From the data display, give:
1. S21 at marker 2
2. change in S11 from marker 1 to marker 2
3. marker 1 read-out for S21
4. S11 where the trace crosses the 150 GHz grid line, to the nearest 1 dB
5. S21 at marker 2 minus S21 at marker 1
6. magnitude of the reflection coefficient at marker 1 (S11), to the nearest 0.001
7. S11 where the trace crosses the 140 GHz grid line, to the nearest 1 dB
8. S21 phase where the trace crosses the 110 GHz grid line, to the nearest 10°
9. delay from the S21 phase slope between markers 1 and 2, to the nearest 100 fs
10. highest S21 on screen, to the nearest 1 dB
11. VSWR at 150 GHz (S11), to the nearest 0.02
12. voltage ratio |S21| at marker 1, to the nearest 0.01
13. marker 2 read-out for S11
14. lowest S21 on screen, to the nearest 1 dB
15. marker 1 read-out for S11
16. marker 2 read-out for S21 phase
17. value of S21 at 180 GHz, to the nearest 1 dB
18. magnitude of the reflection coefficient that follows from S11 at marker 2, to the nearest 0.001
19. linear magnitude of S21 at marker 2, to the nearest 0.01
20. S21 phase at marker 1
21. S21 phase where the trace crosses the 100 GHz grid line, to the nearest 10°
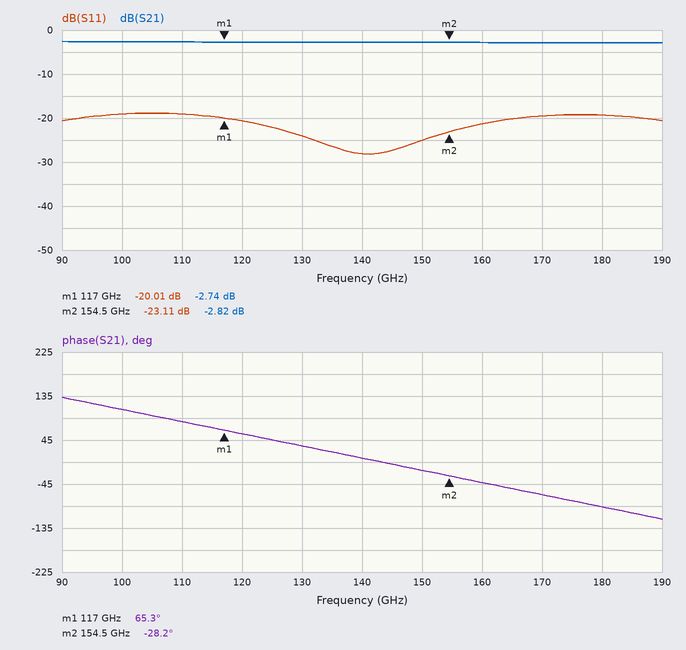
-2.82 dB
-3.10 dB
-2.74 dB
-25 dB
-0.08 dB
0.100
-28 dB
80°
6.9 ps
-3 dB
1.12
0.73
-23.11 dB
-3 dB
-20.01 dB
-28.2°
-3 dB
0.070
0.72
65.3°
110°
